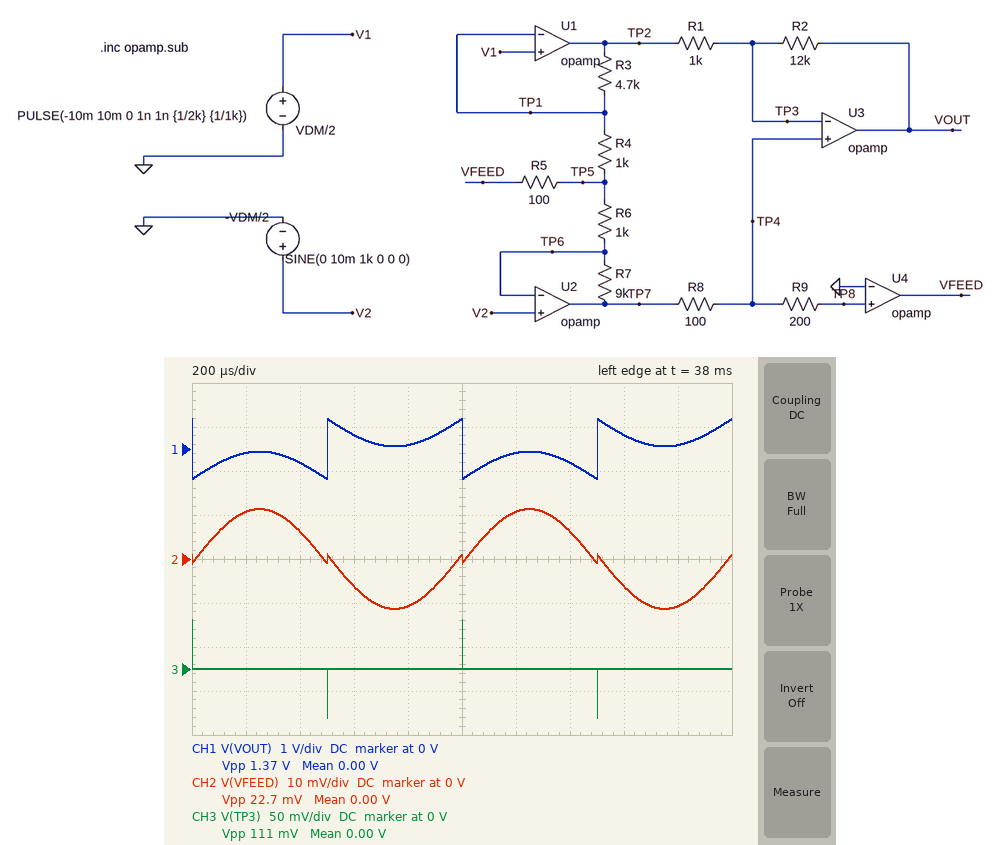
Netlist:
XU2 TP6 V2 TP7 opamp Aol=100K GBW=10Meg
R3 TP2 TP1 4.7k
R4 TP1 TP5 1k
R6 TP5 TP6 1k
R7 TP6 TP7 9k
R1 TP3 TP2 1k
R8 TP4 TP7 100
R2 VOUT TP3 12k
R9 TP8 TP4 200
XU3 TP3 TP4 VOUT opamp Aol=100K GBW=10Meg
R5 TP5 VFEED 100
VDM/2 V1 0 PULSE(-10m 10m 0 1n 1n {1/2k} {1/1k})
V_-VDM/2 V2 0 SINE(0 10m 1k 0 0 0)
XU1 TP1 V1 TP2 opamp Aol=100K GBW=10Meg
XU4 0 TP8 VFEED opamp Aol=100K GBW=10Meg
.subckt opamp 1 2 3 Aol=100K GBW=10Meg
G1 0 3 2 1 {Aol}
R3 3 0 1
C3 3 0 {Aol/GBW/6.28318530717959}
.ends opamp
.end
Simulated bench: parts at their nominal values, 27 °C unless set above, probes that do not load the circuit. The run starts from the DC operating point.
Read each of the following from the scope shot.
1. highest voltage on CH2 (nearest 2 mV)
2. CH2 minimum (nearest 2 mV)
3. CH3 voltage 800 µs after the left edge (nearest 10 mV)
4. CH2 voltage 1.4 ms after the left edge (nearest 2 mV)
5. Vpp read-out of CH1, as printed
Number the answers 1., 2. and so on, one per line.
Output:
1. 12 mV
2. -12 mV
3. 0 V
4. 6 mV
5. 1.37 V
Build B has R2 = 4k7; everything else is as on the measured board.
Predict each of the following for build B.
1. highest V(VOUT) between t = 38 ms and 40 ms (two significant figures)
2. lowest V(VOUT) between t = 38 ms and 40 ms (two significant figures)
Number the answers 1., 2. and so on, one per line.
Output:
1. 270 mV
2. -270 mV
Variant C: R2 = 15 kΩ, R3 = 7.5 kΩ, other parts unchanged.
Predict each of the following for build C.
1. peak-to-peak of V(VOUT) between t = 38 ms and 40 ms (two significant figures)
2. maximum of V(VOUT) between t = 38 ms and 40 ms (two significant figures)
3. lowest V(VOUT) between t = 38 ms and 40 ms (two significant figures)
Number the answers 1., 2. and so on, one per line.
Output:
1. 2.5 V
2. 1.3 V
3. -1.3 V
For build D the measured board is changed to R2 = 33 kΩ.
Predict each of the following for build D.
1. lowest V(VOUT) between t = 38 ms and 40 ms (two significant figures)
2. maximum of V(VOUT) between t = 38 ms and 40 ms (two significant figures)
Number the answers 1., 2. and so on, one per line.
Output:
1. -1.9 V
2. 1.9 V
